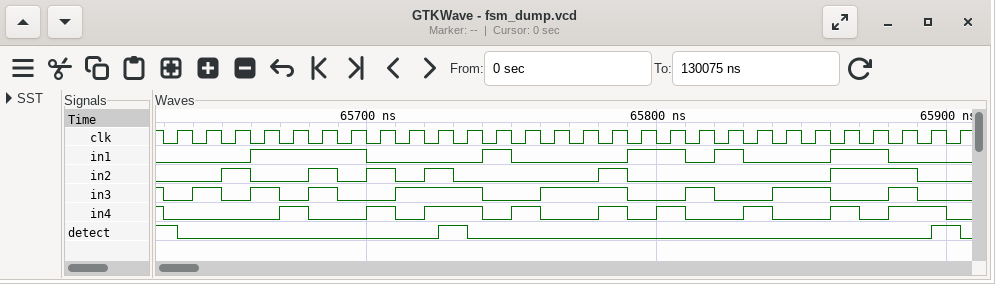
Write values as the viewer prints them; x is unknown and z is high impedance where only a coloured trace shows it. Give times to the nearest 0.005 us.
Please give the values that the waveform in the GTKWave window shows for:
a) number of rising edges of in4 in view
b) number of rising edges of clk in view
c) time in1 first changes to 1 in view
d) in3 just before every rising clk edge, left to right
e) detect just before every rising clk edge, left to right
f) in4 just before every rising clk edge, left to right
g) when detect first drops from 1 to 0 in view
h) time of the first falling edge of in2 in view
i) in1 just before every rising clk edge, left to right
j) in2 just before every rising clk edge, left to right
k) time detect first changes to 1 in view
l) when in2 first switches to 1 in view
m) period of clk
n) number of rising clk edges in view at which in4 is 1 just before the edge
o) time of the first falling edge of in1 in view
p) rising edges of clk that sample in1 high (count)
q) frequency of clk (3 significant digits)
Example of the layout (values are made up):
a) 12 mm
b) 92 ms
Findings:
a) 9
b) 28
c) 65.66 us
d) 0 1 0 1 0 1 0 0 1 1 1 0 0 1 1 1 0 0 1 0 0 1 1 0 0 1 0 0
e) 1 0 0 0 0 0 0 0 0 0 1 0 0 0 0 0 0 0 0 0 0 0 0 0 0 0 0 1
f) 0 0 0 0 1 0 0 1 0 1 1 0 1 0 0 1 0 1 0 0 1 0 0 1 0 1 1 0
g) 65.635 us
h) 65.66 us
i) 0 0 0 1 1 1 1 0 0 0 0 1 0 0 0 0 1 1 0 1 0 0 0 1 1 0 0 0
j) 0 0 1 0 0 1 0 1 0 1 0 0 0 0 0 1 0 0 0 0 0 0 0 1 1 1 0 0
k) 65.725 us
l) 65.65 us
m) 0.01 us
n) 11
o) 65.7 us
p) 10
q) 100 MHz
